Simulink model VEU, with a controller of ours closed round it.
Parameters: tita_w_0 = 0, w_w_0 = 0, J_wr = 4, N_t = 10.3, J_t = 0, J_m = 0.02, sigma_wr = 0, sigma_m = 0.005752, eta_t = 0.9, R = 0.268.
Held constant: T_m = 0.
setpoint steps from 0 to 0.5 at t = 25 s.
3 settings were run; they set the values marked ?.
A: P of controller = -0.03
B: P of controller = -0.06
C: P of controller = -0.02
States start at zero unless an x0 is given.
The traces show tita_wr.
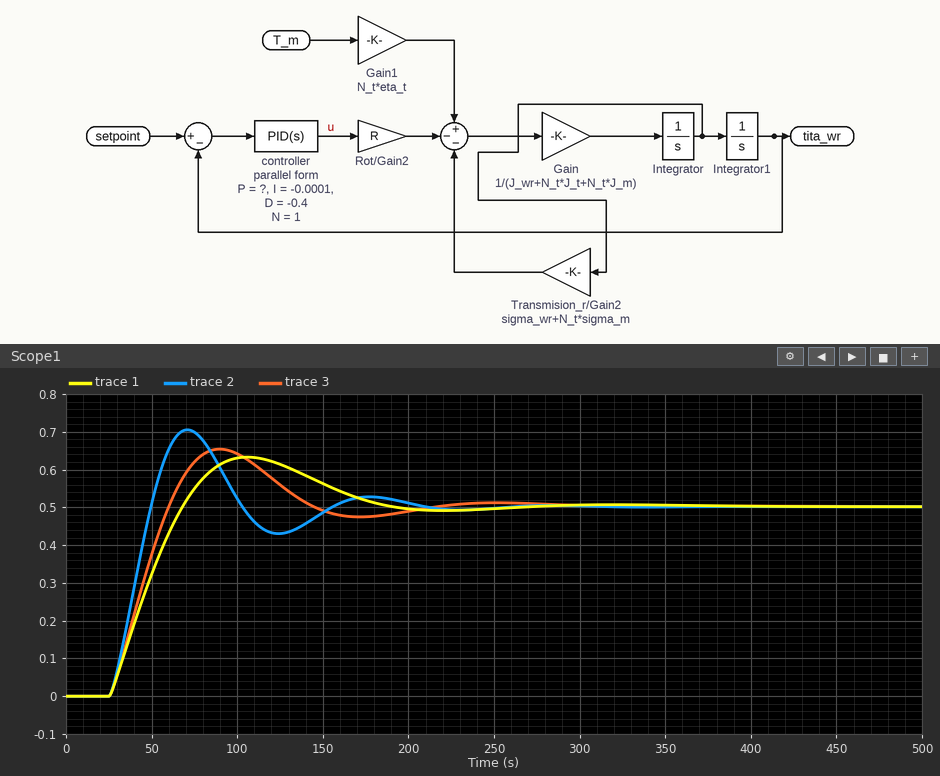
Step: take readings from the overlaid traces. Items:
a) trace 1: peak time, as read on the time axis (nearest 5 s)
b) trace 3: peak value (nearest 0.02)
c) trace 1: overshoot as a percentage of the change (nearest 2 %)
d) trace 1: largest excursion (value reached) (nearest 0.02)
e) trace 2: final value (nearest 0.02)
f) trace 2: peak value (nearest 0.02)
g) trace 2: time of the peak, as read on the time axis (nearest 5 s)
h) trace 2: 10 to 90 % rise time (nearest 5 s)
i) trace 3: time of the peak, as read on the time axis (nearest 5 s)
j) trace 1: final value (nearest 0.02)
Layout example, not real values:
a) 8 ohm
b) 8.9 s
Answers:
a) 105 s
b) 0.66
c) 26 %
d) 0.64
e) 0.50
f) 0.70
g) 70 s
h) 20 s
i) 90 s
j) 0.50
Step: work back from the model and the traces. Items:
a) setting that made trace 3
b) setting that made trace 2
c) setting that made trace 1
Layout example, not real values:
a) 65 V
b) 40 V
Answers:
a) A
b) B
c) C
